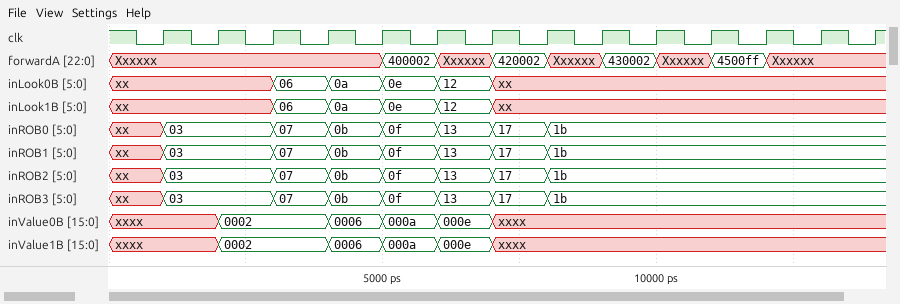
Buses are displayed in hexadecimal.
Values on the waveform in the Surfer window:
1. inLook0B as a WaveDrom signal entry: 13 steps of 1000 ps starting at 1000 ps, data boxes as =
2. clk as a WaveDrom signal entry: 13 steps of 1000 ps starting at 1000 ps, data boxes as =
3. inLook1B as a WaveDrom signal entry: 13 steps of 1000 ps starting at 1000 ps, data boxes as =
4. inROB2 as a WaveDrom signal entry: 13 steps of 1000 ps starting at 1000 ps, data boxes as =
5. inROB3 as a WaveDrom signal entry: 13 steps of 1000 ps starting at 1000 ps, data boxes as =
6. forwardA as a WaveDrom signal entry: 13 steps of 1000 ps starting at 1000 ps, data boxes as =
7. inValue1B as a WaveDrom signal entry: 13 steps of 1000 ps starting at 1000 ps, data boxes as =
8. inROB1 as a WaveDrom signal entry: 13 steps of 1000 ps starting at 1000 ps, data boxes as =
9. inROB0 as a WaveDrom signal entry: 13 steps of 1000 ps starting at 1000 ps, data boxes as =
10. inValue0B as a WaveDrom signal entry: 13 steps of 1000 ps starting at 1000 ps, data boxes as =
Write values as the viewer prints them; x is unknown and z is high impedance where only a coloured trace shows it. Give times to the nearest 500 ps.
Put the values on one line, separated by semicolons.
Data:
{name: 'inLook0B', wave: 'x.====x......', data: '06 0a 0e 12'}; {name: 'clk', wave: 'p............'}; {name: 'inLook1B', wave: 'x.====x......', data: '06 0a 0e 12'}; {name: 'inROB2', wave: '=.======.....', data: '03 07 0b 0f 13 17 1b'}; {name: 'inROB3', wave: '=.======.....', data: '03 07 0b 0f 13 17 1b'}; {name: 'forwardA', wave: '=...========.', data: 'Xxxxxx 400002 Xxxxxx 420002 Xxxxxx 430002 Xxxxxx 4500ff Xxxxxx'}; {name: 'inValue1B', wave: 'x=.===x......', data: '0002 0006 000a 000e'}; {name: 'inROB1', wave: '=.======.....', data: '03 07 0b 0f 13 17 1b'}; {name: 'inROB0', wave: '=.======.....', data: '03 07 0b 0f 13 17 1b'}; {name: 'inValue0B', wave: 'x=.===x......', data: '0002 0006 000a 000e'}
